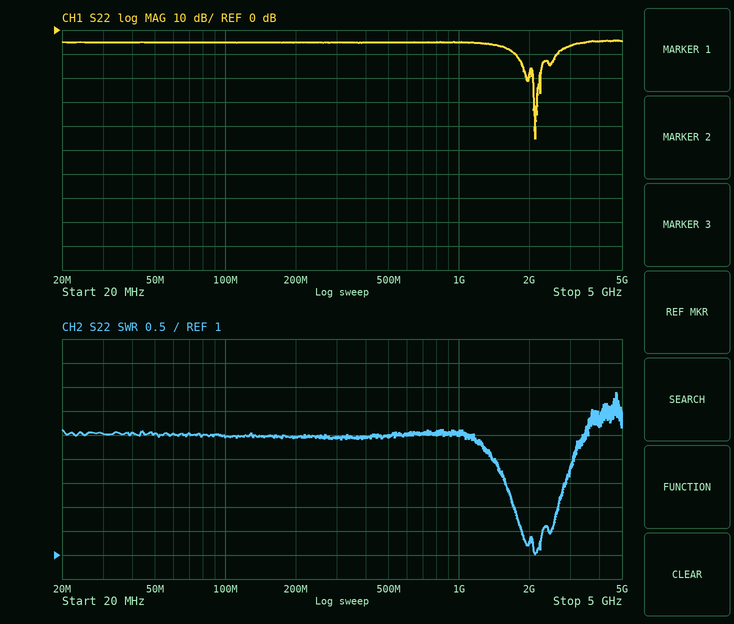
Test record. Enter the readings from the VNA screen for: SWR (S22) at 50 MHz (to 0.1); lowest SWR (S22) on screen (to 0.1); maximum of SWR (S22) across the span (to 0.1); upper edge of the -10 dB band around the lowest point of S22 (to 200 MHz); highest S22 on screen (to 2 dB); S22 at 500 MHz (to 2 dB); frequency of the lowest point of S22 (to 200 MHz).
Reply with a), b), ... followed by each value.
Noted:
a) 3.5
b) 1.0
c) 4.4
d) 2.6 GHz
e) -4 dB
f) -6 dB
g) 2.2 GHz
